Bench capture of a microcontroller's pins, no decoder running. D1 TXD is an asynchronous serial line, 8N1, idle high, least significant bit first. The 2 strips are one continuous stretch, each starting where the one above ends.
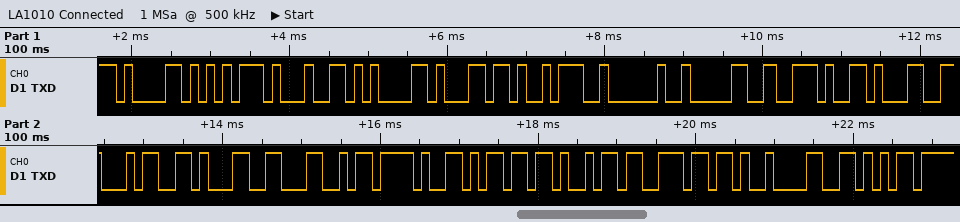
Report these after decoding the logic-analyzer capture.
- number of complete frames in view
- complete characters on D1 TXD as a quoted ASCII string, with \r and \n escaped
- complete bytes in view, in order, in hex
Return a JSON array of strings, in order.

["19", "\"audal: 0.141L/min\\tV\"", "61 75 64 61 6C 3A 20 30 2E 31 34 31 4C 2F 6D 69 6E 09 56"]
